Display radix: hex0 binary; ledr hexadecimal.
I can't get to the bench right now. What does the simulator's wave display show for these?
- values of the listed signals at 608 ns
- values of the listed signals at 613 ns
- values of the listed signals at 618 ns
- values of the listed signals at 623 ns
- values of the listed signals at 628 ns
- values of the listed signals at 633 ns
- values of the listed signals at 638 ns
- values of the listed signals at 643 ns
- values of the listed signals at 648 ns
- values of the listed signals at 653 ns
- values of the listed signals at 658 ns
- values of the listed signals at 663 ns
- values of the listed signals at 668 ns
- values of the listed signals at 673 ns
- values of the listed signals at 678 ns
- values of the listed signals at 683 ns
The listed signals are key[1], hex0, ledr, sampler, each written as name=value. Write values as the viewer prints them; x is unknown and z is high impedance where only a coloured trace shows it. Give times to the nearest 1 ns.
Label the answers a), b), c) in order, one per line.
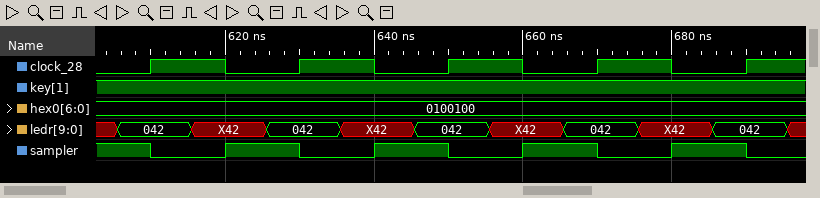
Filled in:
a) key[1]=1, hex0=0100100, ledr=042, sampler=1
b) key[1]=1, hex0=0100100, ledr=042, sampler=0
c) key[1]=1, hex0=0100100, ledr=X42, sampler=0
d) key[1]=1, hex0=0100100, ledr=X42, sampler=1
e) key[1]=1, hex0=0100100, ledr=042, sampler=1
f) key[1]=1, hex0=0100100, ledr=042, sampler=0
g) key[1]=1, hex0=0100100, ledr=X42, sampler=0
h) key[1]=1, hex0=0100100, ledr=X42, sampler=1
i) key[1]=1, hex0=0100100, ledr=042, sampler=1
j) key[1]=1, hex0=0100100, ledr=042, sampler=0
k) key[1]=1, hex0=0100100, ledr=X42, sampler=0
l) key[1]=1, hex0=0100100, ledr=X42, sampler=1
m) key[1]=1, hex0=0100100, ledr=042, sampler=1
n) key[1]=1, hex0=0100100, ledr=042, sampler=0
o) key[1]=1, hex0=0100100, ledr=X42, sampler=0
p) key[1]=1, hex0=0100100, ledr=X42, sampler=1
